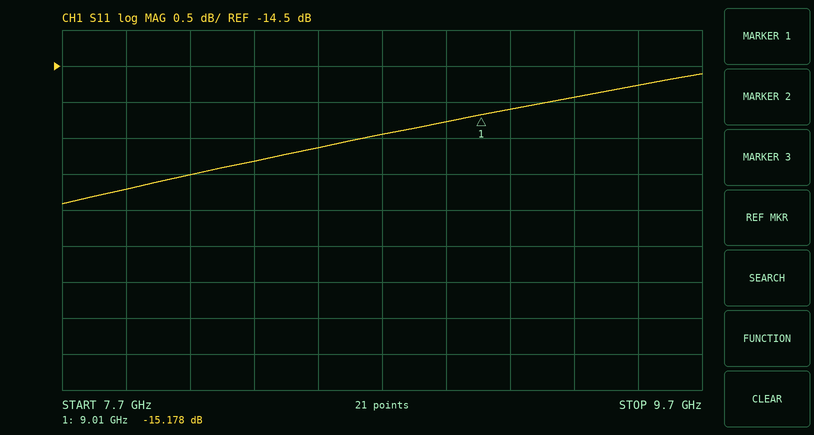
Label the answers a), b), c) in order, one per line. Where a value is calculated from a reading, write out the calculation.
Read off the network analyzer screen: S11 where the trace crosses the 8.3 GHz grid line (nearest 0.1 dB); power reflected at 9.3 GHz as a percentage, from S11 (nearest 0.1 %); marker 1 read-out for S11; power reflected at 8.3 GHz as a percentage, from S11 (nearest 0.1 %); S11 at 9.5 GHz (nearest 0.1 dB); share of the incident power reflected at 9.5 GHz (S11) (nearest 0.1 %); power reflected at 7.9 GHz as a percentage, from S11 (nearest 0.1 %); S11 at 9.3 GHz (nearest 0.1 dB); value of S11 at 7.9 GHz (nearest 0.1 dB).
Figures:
a) -15.8 dB
b) 10^(-14.9/10) ≈ 3.2 %
c) -15.178 dB
d) 10^(-15.8/10) ≈ 2.6 %
e) -14.8 dB
f) 10^(-14.8/10) ≈ 3.3 %
g) 10^(-16.2/10) ≈ 2.4 %
h) -14.9 dB
i) -16.2 dB
